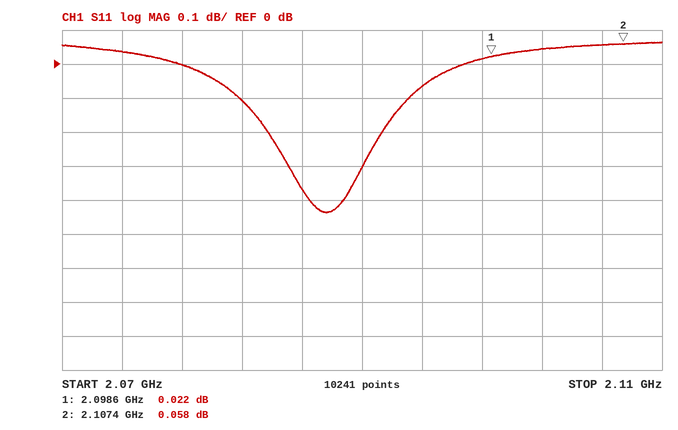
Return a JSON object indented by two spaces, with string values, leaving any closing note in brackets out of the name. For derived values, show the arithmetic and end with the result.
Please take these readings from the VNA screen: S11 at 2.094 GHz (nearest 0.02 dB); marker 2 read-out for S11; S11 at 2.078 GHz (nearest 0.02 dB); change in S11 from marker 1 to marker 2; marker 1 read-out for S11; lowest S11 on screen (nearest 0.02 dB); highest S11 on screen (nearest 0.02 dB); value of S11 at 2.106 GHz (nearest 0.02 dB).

{
  "S11 at 2.094 GHz": "-0.06 dB",
  "marker 2 read-out for S11": "0.058 dB",
  "S11 at 2.078 GHz": "0.00 dB",
  "change in S11 from marker 1 to marker 2": "0.058 − (0.022) = 0.036 dB",
  "marker 1 read-out for S11": "0.022 dB",
  "lowest S11 on screen": "-0.44 dB",
  "highest S11 on screen": "0.06 dB",
  "value of S11 at 2.106 GHz": "0.06 dB"
}
